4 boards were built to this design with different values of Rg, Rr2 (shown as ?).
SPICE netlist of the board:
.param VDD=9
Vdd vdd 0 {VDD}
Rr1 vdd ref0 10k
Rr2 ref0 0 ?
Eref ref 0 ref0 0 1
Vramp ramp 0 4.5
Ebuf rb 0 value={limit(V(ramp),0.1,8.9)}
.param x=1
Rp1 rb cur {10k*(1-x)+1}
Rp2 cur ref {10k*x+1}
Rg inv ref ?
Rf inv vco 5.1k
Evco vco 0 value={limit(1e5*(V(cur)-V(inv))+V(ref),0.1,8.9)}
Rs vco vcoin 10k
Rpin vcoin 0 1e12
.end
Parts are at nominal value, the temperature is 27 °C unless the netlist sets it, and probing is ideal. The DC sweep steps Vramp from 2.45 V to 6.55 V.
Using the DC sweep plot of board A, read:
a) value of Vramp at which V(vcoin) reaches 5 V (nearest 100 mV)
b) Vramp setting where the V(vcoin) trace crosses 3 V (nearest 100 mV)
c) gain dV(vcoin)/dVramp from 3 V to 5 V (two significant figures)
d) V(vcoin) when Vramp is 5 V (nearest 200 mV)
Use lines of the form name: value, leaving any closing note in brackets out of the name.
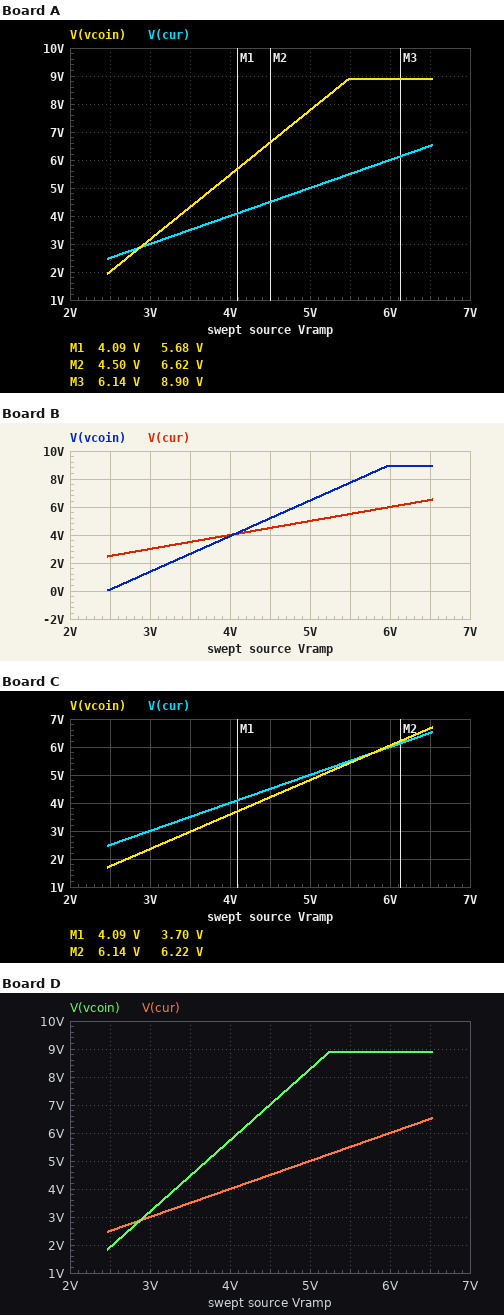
value of Vramp at which V(vcoin) reaches 5 V: 3.8 V
Vramp setting where the V(vcoin) trace crosses 3 V: 2.9 V
gain dV(vcoin)/dVramp from 3 V to 5 V: 2.3 V/V
V(vcoin) when Vramp is 5 V: 7.8 V
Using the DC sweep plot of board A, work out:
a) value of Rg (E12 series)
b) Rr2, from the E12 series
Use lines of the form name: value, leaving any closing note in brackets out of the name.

value of Rg: 3.9 kΩ
Rr2, from the E12 series: 4.7 kΩ
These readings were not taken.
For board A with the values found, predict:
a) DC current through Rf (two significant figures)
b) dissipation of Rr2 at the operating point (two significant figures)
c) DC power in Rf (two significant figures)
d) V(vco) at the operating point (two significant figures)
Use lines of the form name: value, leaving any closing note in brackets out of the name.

DC current through Rf: 420 µA
dissipation of Rr2 at the operating point: 1.8 mW
DC power in Rf: 880 µW
V(vco) at the operating point: 6.6 V
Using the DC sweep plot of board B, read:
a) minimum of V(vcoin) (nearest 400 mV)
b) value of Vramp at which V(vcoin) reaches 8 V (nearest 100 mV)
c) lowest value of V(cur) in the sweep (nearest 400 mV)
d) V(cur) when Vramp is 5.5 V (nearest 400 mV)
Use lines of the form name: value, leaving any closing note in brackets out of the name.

minimum of V(vcoin): 0 V
value of Vramp at which V(vcoin) reaches 8 V: 5.6 V
lowest value of V(cur) in the sweep: 2.4 V
V(cur) when Vramp is 5.5 V: 5.6 V
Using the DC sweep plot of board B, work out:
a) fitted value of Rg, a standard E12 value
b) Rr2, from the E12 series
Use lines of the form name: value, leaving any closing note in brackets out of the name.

fitted value of Rg, a standard E12 value: 3.3 kΩ
Rr2, from the E12 series: 8.2 kΩ
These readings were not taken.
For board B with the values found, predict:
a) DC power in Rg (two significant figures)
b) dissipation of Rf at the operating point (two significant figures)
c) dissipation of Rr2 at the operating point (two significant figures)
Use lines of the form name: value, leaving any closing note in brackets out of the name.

DC power in Rg: 60 µW
dissipation of Rf at the operating point: 93 µW
dissipation of Rr2 at the operating point: 2.0 mW
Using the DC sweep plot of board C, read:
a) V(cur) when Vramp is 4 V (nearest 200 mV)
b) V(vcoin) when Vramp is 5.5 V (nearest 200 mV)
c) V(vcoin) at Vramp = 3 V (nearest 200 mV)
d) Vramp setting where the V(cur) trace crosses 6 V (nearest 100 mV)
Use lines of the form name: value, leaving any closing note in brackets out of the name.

V(cur) when Vramp is 4 V: 4.0 V
V(vcoin) when Vramp is 5.5 V: 5.4 V
V(vcoin) at Vramp = 3 V: 2.4 V
Vramp setting where the V(cur) trace crosses 6 V: 6.0 V
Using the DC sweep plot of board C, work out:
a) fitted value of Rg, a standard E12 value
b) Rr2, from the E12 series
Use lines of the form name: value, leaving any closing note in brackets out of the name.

fitted value of Rg, a standard E12 value: 22 kΩ
Rr2, from the E12 series: 18 kΩ
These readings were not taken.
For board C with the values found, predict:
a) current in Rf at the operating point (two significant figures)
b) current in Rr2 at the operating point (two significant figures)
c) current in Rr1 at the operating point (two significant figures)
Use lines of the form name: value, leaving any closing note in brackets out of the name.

current in Rf at the operating point: 58 µA
current in Rr2 at the operating point: 320 µA
current in Rr1 at the operating point: 320 µA
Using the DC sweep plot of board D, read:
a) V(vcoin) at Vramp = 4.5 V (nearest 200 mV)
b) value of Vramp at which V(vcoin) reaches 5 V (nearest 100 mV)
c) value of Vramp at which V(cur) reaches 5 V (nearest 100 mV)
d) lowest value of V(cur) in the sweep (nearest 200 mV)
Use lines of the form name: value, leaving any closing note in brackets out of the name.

V(vcoin) at Vramp = 4.5 V: 7.0 V
value of Vramp at which V(vcoin) reaches 5 V: 3.7 V
value of Vramp at which V(cur) reaches 5 V: 5.0 V
lowest value of V(cur) in the sweep: 2.4 V
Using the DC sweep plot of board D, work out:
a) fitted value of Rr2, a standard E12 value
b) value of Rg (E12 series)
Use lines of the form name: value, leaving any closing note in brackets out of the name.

fitted value of Rr2, a standard E12 value: 4.7 kΩ
value of Rg: 3.3 kΩ
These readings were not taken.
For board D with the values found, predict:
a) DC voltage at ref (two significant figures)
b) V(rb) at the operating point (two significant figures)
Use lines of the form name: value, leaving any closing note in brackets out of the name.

DC voltage at ref: 2.9 V
V(rb) at the operating point: 4.5 V
